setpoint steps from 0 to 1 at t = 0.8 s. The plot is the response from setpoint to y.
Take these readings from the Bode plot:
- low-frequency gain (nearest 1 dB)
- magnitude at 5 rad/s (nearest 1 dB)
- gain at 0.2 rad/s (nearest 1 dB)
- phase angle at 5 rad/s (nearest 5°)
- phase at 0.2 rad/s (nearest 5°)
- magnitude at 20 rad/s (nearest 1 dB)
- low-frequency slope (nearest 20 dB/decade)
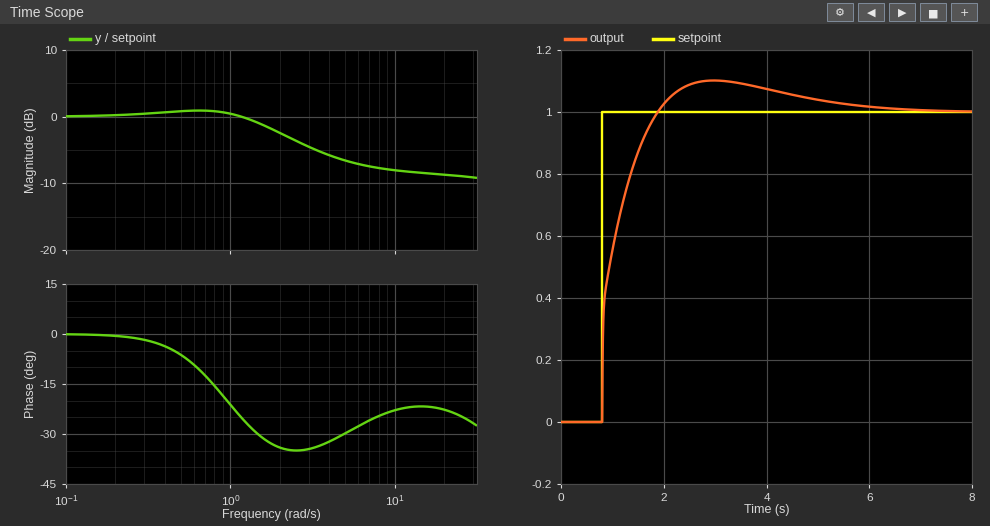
0 dB
-7 dB
0 dB
-30°
0°
-9 dB
0 dB/decade
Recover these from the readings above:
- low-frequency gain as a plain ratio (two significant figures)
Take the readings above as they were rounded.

1.0
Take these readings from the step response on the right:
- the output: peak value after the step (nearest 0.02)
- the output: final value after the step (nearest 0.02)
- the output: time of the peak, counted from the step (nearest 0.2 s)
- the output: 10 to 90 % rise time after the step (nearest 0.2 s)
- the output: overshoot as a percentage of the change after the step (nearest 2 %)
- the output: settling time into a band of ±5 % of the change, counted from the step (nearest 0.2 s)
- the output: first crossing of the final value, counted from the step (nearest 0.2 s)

1.10
1.00
2.2 s
0.8 s
10 %
3.8 s
1.0 s
